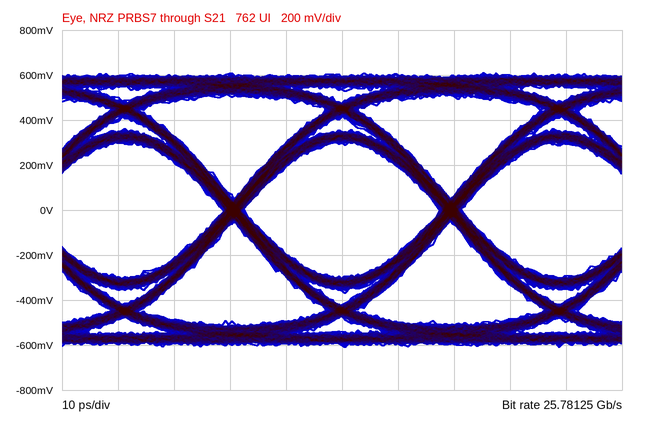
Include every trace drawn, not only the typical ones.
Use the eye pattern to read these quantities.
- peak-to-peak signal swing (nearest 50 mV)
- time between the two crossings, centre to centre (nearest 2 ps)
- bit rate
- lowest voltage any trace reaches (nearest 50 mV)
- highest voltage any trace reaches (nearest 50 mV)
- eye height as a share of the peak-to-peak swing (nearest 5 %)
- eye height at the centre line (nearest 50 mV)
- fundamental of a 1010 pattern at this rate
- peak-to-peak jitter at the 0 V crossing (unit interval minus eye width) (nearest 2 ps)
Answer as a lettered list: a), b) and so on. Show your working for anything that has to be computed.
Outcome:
a) 1.20 V
b) 38 ps
c) 25.78125 Gb/s
d) -600 mV
e) 600 mV
f) 600 mV / 1.20 V ≈ 50 %
g) 600 mV
h) 12.89062 GHz
i) 4 ps
